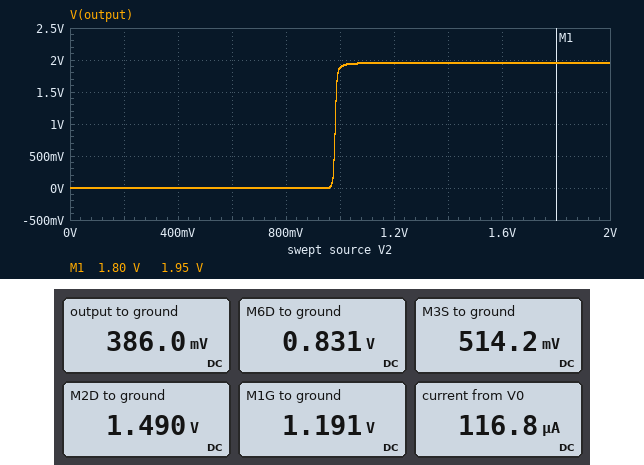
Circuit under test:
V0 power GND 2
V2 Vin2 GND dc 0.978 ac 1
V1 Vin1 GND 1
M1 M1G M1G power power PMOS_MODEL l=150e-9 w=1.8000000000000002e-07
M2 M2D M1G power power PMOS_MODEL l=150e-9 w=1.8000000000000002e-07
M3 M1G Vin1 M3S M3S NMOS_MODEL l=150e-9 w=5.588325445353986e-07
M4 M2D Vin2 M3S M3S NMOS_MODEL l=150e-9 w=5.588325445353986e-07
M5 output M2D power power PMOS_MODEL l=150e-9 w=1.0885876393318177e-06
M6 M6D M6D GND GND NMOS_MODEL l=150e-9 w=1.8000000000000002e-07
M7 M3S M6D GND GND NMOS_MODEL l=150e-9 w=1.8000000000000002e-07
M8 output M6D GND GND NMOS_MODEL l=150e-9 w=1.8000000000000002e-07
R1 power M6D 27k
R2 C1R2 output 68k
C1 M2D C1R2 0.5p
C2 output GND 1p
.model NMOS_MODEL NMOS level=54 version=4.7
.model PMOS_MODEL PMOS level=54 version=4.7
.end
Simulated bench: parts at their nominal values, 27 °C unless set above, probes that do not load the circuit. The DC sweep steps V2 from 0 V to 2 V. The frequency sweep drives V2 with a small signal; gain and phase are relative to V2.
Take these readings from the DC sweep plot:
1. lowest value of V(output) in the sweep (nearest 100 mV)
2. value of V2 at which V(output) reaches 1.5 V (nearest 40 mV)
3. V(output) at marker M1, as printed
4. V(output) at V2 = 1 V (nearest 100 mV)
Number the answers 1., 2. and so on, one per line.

1. 0 V
2. 1.00 V
3. 1.95 V
4. 1.9 V
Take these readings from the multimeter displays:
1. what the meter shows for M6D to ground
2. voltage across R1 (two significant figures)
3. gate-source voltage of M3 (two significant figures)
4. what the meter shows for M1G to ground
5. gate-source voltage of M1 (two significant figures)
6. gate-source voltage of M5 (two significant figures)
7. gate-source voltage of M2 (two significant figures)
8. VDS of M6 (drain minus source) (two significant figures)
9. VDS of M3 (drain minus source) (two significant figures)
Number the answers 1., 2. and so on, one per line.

1. 0.831 V
2. 1.2 V
3. 490 mV
4. 1.191 V
5. -810 mV
6. -510 mV
7. -810 mV
8. 830 mV
9. 680 mV
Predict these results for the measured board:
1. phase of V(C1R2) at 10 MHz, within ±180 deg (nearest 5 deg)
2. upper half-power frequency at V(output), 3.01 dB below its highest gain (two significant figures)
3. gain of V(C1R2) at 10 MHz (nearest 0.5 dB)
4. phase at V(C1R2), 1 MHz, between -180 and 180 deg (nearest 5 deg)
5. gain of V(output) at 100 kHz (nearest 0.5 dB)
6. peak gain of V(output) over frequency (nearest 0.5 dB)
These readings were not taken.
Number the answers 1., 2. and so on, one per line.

1. -120 deg
2. 470 kHz
3. 16.5 dB
4. -70 deg
5. 40.0 dB
6. 40.0 dB
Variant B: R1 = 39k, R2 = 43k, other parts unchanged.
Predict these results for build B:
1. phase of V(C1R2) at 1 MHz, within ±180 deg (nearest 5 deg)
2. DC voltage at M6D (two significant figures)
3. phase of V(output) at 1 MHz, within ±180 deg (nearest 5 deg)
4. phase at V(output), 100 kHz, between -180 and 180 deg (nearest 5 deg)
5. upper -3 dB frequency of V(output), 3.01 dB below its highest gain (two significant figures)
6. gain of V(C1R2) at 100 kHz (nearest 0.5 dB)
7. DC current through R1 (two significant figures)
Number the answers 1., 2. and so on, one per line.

1. -45 deg
2. 740 mV
3. -35 deg
4. -5 deg
5. 1.2 MHz
6. 28.5 dB
7. 32 µA
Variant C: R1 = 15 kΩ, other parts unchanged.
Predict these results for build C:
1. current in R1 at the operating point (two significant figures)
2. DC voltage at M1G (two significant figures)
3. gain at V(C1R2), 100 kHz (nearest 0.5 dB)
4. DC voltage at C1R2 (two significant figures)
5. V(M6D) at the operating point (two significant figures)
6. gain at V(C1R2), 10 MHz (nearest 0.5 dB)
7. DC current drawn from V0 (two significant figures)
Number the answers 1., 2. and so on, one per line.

1. 67 µA
2. 1.1 V
3. 39.0 dB
4. 1.3 V
5. 1.0 V
6. 17.0 dB
7. 190 µA
